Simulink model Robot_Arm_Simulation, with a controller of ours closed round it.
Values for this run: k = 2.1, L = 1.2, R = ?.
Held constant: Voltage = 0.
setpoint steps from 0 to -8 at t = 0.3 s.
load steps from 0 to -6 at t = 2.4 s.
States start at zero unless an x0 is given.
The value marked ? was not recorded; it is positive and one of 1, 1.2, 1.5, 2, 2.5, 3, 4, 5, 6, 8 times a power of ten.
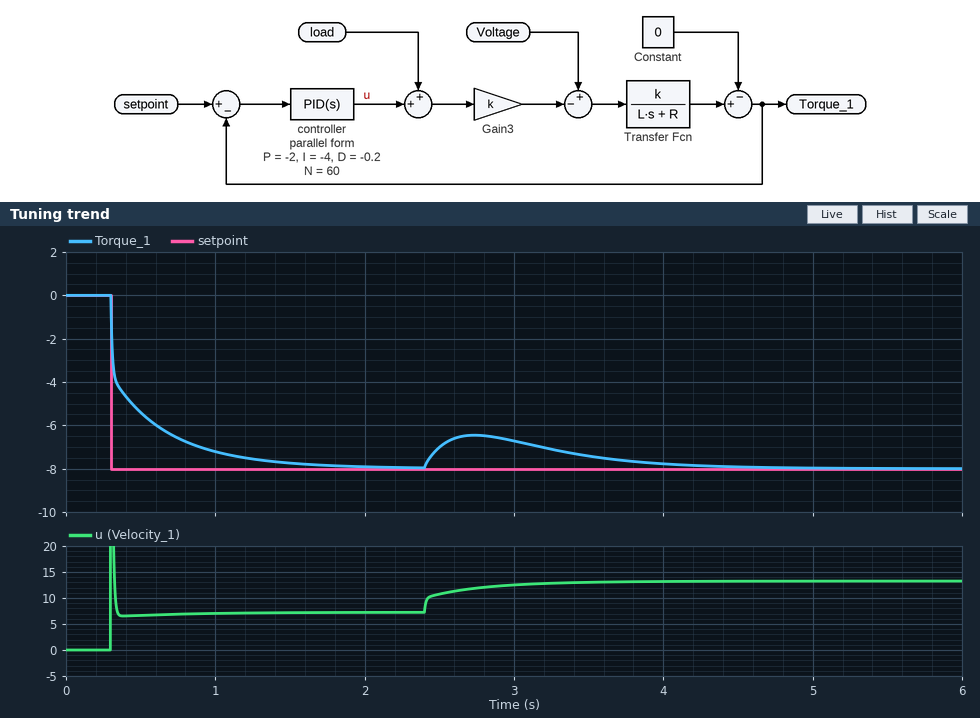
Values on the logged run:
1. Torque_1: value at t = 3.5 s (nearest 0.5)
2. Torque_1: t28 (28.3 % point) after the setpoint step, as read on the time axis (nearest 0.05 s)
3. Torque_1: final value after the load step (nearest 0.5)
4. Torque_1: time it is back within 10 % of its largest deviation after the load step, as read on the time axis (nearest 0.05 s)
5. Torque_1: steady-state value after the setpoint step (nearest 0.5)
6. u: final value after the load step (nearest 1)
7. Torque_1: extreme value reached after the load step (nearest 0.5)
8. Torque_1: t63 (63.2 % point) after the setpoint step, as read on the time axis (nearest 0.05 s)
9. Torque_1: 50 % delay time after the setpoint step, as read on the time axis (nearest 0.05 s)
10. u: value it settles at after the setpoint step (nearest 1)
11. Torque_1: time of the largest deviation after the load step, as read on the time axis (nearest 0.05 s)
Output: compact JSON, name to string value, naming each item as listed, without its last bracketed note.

{"Torque_1: value at t = 3.5 s": "-7.5", "Torque_1: t28 (28.3 % point) after the setpoint step, as read on the time axis": "0.30 s", "Torque_1: final value after the load step": "-8.0", "Torque_1: time it is back within 10 % of its largest deviation after the load step, as read on the time axis": "4.20 s", "Torque_1: steady-state value after the setpoint step": "-8.0", "u: final value after the load step": "13", "Torque_1: extreme value reached after the load step": "-6.5", "Torque_1: t63 (63.2 % point) after the setpoint step, as read on the time axis": "0.45 s", "Torque_1: 50 % delay time after the setpoint step, as read on the time axis": "0.35 s", "u: value it settles at after the setpoint step": "7", "Torque_1: time of the largest deviation after the load step, as read on the time axis": "2.75 s"}
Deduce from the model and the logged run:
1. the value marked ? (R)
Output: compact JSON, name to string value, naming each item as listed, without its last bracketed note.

{"the value marked ?": "4"}
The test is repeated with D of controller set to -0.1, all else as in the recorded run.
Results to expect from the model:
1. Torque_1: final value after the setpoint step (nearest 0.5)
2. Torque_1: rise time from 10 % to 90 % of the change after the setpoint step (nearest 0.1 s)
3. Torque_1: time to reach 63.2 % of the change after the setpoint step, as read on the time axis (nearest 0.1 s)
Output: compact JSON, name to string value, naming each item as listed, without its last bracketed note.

{"Torque_1: final value after the setpoint step": "-8.0", "Torque_1: rise time from 10 % to 90 % of the change after the setpoint step": "0.6 s", "Torque_1: time to reach 63.2 % of the change after the setpoint step, as read on the time axis": "0.5 s"}
